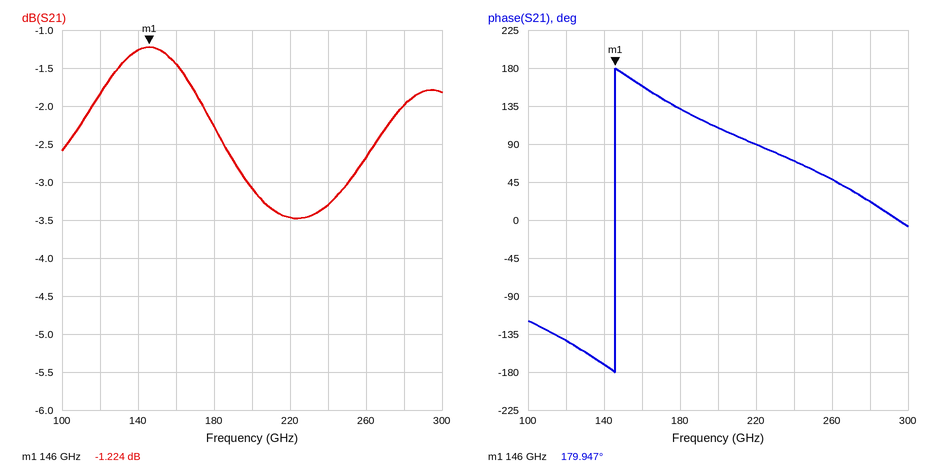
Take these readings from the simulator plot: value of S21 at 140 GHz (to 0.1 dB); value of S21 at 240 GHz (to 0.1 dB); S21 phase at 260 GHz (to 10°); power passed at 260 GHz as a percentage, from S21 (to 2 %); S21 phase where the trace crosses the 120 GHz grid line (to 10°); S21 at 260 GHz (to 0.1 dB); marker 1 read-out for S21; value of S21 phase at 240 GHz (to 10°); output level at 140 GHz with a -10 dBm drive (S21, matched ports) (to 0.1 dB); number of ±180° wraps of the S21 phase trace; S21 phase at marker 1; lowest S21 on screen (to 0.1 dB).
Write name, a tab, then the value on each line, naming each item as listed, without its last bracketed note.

value of S21 at 140 GHz	-1.3 dB
value of S21 at 240 GHz	-3.3 dB
S21 phase at 260 GHz	50°
power passed at 260 GHz as a percentage, from S21	54 %
S21 phase where the trace crosses the 120 GHz grid line	-140°
S21 at 260 GHz	-2.7 dB
marker 1 read-out for S21	-1.224 dB
value of S21 phase at 240 GHz	70°
output level at 140 GHz with a -10 dBm drive (S21, matched ports)	-11.3 dBm
number of ±180° wraps of the S21 phase trace	1
S21 phase at marker 1	179.947°
lowest S21 on screen	-3.5 dB
